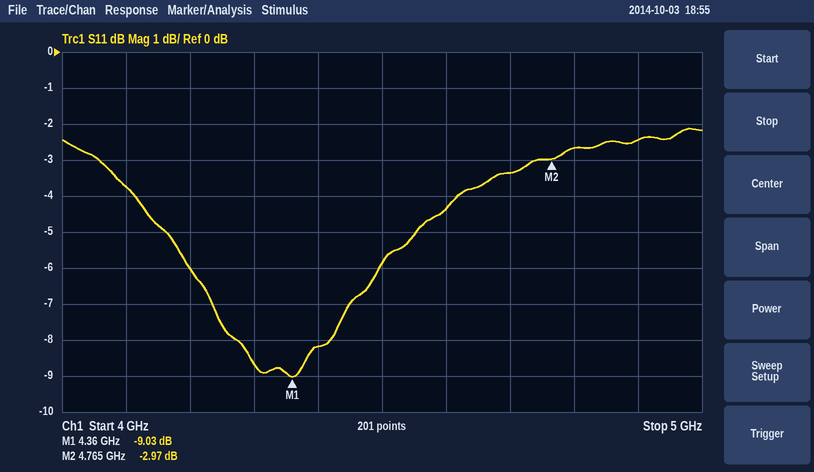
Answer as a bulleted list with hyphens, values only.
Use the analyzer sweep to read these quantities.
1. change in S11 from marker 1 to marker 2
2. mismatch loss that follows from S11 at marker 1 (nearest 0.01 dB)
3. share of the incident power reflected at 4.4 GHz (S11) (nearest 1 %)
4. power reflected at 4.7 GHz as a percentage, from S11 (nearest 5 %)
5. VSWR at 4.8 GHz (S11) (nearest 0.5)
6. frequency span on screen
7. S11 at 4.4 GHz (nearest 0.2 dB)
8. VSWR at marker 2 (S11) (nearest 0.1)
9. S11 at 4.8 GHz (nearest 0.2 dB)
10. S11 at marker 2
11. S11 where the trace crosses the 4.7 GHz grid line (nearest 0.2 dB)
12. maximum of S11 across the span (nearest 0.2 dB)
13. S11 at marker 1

- 6.06 dB
- 0.58 dB
- 15 %
- 45 %
- 6.5
- 1 GHz
- -8.2 dB
- 5.9
- -2.6 dB
- -2.97 dB
- -3.4 dB
- -2.2 dB
- -9.03 dB
